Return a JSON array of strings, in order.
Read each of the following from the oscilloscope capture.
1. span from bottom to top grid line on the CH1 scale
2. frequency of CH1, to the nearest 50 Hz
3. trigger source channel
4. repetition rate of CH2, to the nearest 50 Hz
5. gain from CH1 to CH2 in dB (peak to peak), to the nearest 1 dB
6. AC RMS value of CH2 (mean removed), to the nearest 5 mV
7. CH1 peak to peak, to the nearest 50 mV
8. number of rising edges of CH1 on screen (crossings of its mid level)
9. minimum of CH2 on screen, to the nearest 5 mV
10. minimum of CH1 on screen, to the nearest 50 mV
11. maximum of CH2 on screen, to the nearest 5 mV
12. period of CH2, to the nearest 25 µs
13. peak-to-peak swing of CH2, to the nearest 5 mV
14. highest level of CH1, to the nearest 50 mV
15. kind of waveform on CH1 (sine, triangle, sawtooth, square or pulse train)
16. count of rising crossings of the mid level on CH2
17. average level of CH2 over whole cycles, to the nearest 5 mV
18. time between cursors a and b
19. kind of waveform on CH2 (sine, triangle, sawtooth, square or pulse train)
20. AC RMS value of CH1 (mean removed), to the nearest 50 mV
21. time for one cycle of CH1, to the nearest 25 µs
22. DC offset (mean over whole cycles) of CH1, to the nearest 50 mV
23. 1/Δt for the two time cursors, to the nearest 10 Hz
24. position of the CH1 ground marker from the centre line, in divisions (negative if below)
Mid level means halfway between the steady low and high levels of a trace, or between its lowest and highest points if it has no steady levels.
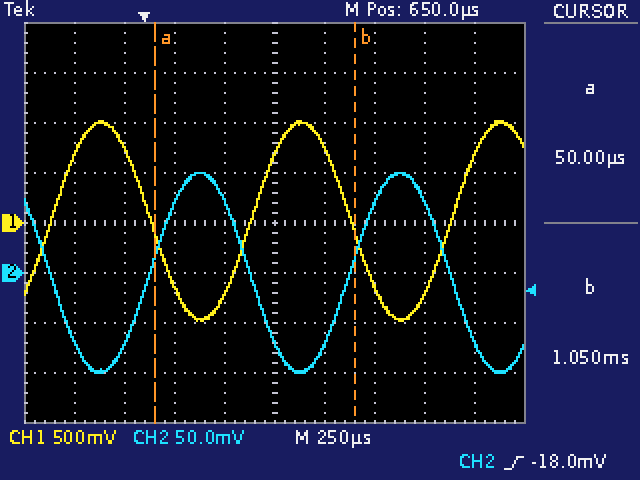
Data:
["4 V", "1.00 kHz", "CH2", "1.00 kHz", "-20 dB", "70 mV", "2.00 V", "3", "-100 mV", "-1.00 V", "100 mV", "1.000 ms", "200 mV", "1.00 V", "sine", "2", "0 mV", "1.000 ms", "sine", "700 mV", "1.000 ms", "0 mV", "1.00 kHz", "0.0 div"]
